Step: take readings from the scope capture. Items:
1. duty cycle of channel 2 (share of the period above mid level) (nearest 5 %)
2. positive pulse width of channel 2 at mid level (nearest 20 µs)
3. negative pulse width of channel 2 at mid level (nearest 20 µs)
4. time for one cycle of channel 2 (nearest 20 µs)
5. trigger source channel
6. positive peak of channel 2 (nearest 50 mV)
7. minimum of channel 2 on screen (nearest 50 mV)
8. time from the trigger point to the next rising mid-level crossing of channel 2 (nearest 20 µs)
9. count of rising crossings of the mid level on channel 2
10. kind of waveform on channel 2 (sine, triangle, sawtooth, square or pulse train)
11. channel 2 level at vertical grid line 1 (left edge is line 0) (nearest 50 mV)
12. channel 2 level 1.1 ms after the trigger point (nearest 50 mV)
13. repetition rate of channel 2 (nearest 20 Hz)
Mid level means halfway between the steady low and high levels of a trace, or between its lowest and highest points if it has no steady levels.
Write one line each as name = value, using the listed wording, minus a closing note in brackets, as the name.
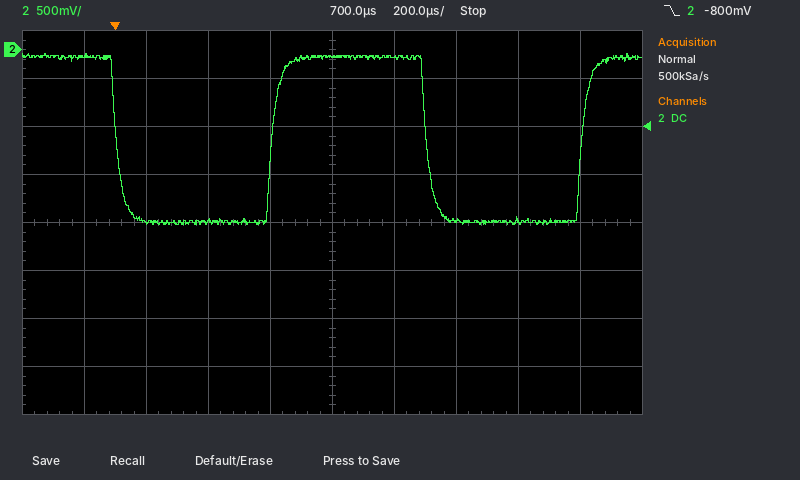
duty cycle of channel 2 (share of the period above mid level) = 50 %
positive pulse width of channel 2 at mid level = 500 µs
negative pulse width of channel 2 at mid level = 500 µs
time for one cycle of channel 2 = 1.00 ms
trigger source channel = channel 2
positive peak of channel 2 = -50 mV
minimum of channel 2 on screen = -1.80 V
time from the trigger point to the next rising mid-level crossing of channel 2 = 500 µs
count of rising crossings of the mid level on channel 2 = 2
kind of waveform on channel 2 = square
channel 2 level at vertical grid line 1 (left edge is line 0) = -50 mV
channel 2 level 1.1 ms after the trigger point = -1.80 V
repetition rate of channel 2 = 1.00 kHz
